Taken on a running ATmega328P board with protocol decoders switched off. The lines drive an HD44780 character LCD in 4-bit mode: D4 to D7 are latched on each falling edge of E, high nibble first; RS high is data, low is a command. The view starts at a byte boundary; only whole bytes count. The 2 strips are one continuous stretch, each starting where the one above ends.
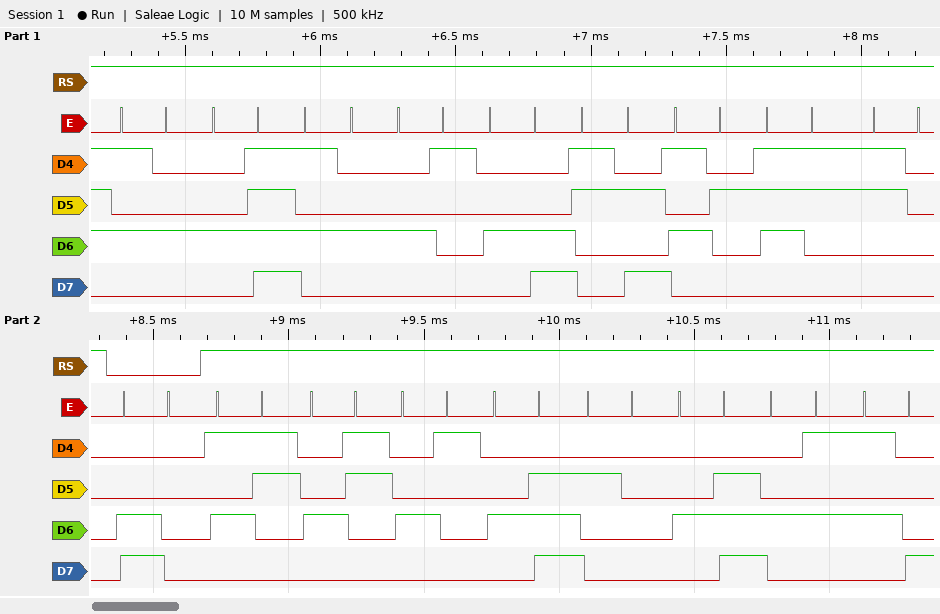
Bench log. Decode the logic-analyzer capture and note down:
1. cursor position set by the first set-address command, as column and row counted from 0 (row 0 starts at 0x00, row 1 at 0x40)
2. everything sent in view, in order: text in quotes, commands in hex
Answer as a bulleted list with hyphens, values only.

- column 0, row 1
- "TOTAL:Rs0" 0xC0 "SCAN NEX"
